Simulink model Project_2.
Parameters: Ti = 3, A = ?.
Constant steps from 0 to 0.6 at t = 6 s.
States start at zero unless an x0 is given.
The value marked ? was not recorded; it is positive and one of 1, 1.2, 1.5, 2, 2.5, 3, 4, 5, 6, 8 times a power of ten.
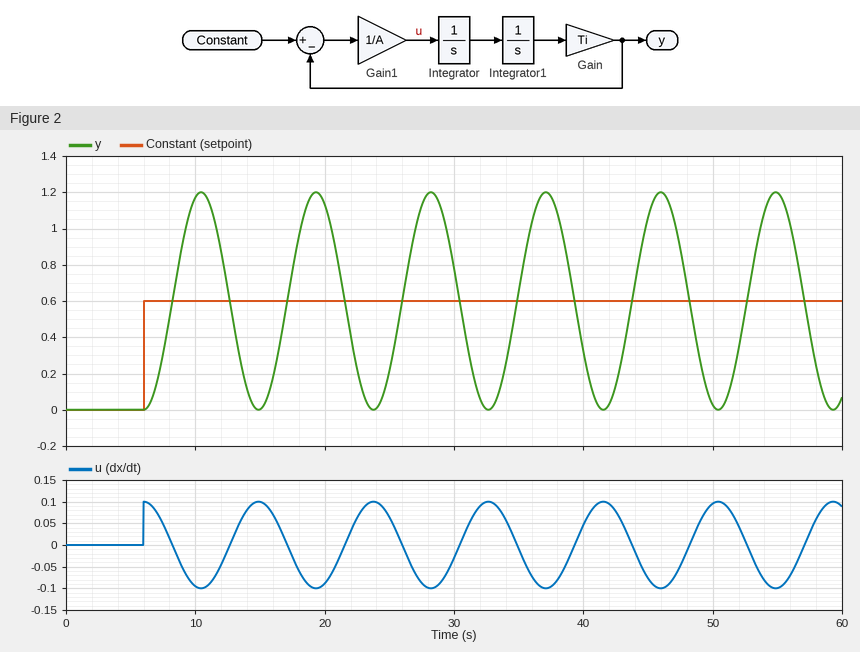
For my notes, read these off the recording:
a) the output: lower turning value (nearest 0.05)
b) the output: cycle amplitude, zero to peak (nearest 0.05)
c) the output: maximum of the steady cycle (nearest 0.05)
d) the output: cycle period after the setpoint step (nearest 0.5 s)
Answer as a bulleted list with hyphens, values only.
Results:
- 0.00
- 0.60
- 1.20
- 9.0 s
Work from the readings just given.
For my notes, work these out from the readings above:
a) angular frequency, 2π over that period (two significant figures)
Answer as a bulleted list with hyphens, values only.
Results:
- 0.70 rad/s
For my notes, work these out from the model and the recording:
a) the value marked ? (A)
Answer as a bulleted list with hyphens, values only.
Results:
- 6
